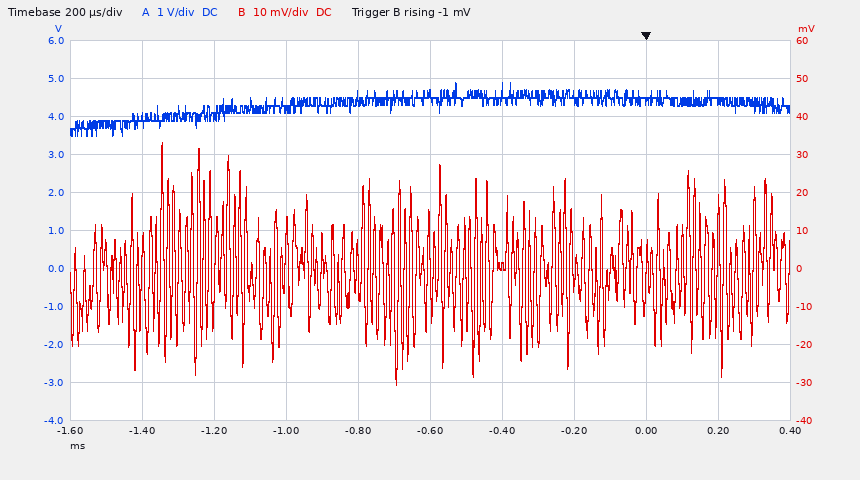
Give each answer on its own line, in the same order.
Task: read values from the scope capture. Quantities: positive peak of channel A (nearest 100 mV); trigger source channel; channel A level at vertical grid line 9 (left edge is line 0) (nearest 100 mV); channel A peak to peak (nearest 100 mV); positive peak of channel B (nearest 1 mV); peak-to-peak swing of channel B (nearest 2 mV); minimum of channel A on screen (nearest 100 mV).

4.9 V
channel B
4.4 V
1.4 V
33 mV
64 mV
3.5 V
